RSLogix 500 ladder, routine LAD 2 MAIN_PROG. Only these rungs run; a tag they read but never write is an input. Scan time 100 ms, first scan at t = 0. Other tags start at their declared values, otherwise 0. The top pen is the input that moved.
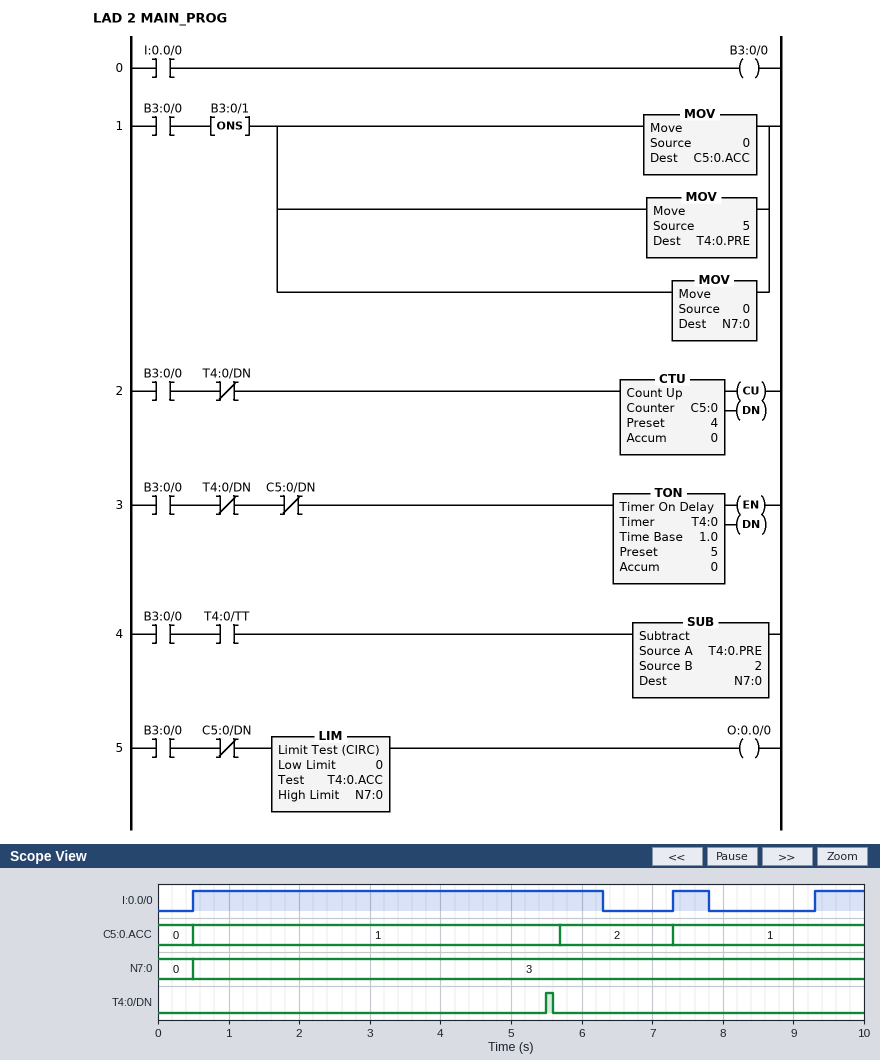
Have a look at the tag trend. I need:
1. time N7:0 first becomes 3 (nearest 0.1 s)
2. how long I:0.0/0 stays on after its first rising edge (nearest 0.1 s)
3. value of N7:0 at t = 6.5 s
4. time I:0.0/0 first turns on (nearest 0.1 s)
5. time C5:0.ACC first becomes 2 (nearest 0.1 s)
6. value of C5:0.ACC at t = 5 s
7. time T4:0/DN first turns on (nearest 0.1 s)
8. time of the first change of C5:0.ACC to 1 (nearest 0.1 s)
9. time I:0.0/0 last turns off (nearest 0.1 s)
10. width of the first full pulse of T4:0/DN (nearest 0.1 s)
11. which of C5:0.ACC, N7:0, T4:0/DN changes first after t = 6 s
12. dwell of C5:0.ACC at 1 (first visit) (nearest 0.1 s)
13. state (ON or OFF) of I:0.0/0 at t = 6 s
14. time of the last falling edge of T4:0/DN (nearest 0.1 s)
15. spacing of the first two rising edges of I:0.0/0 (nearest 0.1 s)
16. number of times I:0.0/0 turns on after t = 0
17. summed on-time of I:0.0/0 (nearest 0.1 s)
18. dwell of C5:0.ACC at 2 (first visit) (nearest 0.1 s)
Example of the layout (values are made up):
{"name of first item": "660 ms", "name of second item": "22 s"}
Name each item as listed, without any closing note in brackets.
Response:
{"time N7:0 first becomes 3": "0.5 s", "how long I:0.0/0 stays on after its first rising edge": "5.8 s", "value of N7:0 at t = 6.5 s": "3", "time I:0.0/0 first turns on": "0.5 s", "time C5:0.ACC first becomes 2": "5.7 s", "value of C5:0.ACC at t = 5 s": "1", "time T4:0/DN first turns on": "5.5 s", "time of the first change of C5:0.ACC to 1": "0.5 s", "time I:0.0/0 last turns off": "7.8 s", "width of the first full pulse of T4:0/DN": "0.1 s", "which of C5:0.ACC, N7:0, T4:0/DN changes first after t = 6 s": "C5:0.ACC", "dwell of C5:0.ACC at 1 (first visit)": "5.2 s", "state (ON or OFF) of I:0.0/0 at t = 6 s": "ON", "time of the last falling edge of T4:0/DN": "5.6 s", "spacing of the first two rising edges of I:0.0/0": "6.8 s", "number of times I:0.0/0 turns on after t = 0": "3", "summed on-time of I:0.0/0": "7.0 s", "dwell of C5:0.ACC at 2 (first visit)": "1.6 s"}
